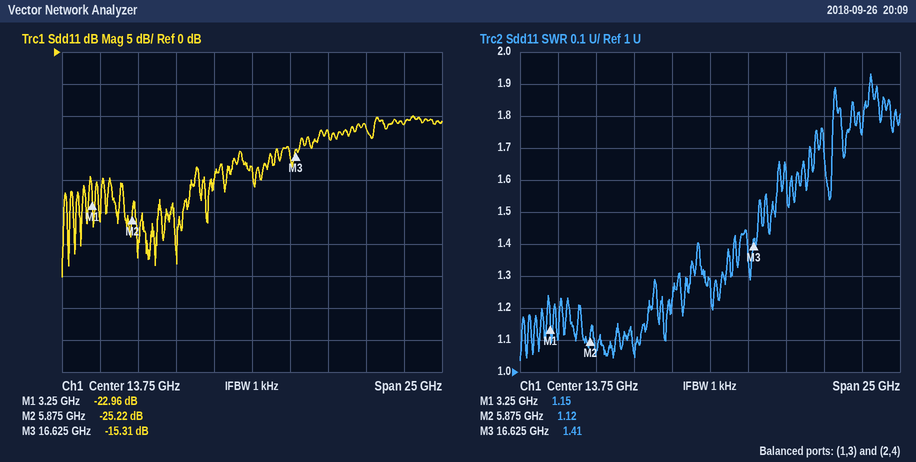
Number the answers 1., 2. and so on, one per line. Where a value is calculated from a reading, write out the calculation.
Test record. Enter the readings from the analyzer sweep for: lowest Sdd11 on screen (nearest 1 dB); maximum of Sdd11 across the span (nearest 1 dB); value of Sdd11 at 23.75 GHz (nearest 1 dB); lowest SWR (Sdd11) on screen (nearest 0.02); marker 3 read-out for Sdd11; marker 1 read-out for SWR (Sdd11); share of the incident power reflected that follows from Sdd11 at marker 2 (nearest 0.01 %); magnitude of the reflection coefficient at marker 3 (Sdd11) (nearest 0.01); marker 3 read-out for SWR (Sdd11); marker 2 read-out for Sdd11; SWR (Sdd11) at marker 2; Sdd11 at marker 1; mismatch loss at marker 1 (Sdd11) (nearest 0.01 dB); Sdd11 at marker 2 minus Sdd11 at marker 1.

1. -35 dB
2. -10 dB
3. -11 dB
4. 1.04
5. -15.31 dB
6. 1.15
7. 10^(-25.22/10) ≈ 0.30 %
8. 10^(-15.31/20) ≈ 0.17
9. 1.41
10. -25.22 dB
11. 1.12
12. -22.96 dB
13. −10 log10(1 − 10^(-22.96/10)) ≈ 0.02 dB
14. -25.22 − (-22.96) = -2.26 dB
